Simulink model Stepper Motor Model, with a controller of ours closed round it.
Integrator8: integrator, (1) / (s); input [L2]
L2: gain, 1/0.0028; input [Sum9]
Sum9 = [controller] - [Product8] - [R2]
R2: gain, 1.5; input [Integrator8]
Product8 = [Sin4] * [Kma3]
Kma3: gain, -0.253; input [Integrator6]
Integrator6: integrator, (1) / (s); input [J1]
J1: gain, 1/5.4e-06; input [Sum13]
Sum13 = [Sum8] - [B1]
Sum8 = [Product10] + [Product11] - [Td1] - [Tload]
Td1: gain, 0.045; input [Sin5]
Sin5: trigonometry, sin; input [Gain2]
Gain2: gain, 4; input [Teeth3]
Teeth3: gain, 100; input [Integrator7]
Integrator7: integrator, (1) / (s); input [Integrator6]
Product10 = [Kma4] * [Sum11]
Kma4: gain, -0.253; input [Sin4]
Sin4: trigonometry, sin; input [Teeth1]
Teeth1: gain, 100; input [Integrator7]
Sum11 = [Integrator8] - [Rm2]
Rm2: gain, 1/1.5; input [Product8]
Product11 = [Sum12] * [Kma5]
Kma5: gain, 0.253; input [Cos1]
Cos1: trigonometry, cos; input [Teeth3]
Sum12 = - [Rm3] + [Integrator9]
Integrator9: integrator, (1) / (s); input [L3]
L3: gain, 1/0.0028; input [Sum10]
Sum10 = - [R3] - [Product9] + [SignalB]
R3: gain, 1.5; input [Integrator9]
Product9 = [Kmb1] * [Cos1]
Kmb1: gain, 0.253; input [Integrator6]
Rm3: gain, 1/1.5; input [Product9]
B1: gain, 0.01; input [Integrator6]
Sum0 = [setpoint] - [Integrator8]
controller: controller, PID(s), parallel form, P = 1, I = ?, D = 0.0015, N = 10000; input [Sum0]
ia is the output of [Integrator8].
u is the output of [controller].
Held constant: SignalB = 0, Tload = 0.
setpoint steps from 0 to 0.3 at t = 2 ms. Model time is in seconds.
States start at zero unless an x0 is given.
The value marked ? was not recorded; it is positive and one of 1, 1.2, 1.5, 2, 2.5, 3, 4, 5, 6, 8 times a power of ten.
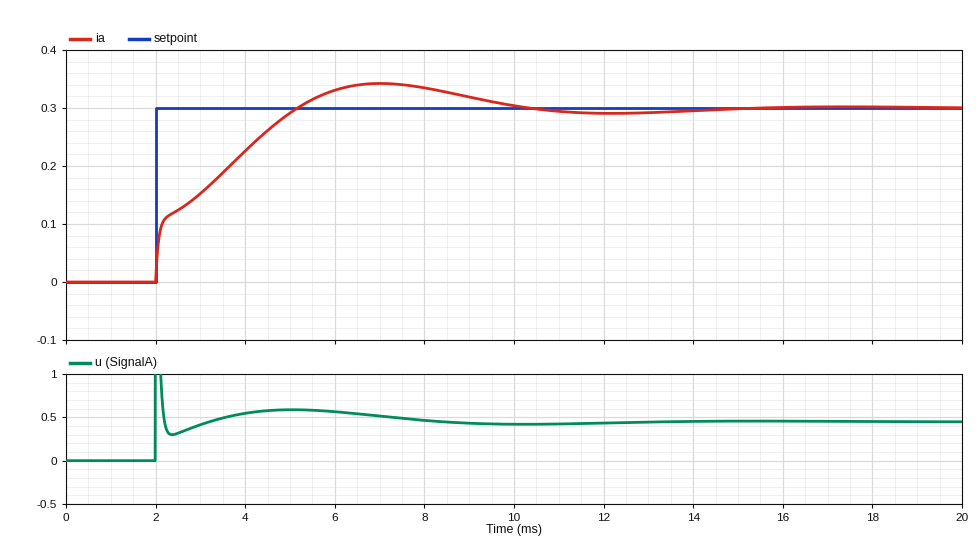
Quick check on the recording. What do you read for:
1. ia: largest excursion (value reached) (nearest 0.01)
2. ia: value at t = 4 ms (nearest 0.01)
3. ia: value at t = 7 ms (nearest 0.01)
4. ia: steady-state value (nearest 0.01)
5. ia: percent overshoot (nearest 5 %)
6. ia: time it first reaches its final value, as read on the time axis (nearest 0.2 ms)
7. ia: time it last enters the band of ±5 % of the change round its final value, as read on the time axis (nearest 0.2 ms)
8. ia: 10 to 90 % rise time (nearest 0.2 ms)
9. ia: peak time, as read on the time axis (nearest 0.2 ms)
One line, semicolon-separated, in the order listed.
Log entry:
0.34; 0.23; 0.34; 0.30; 15 %; 5.2 ms; 9.2 ms; 2.6 ms; 7.0 ms
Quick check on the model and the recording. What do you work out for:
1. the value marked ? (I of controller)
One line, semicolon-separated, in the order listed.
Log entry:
2000
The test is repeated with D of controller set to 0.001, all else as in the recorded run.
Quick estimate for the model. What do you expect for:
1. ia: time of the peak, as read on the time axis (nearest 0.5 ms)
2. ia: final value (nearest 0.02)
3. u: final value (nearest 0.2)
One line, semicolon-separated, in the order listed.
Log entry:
6.5 ms; 0.30; 0.4
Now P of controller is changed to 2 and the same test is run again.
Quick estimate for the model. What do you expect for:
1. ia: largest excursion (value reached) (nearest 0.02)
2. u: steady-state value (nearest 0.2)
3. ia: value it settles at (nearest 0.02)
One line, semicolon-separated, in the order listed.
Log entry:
0.32; 0.4; 0.30
